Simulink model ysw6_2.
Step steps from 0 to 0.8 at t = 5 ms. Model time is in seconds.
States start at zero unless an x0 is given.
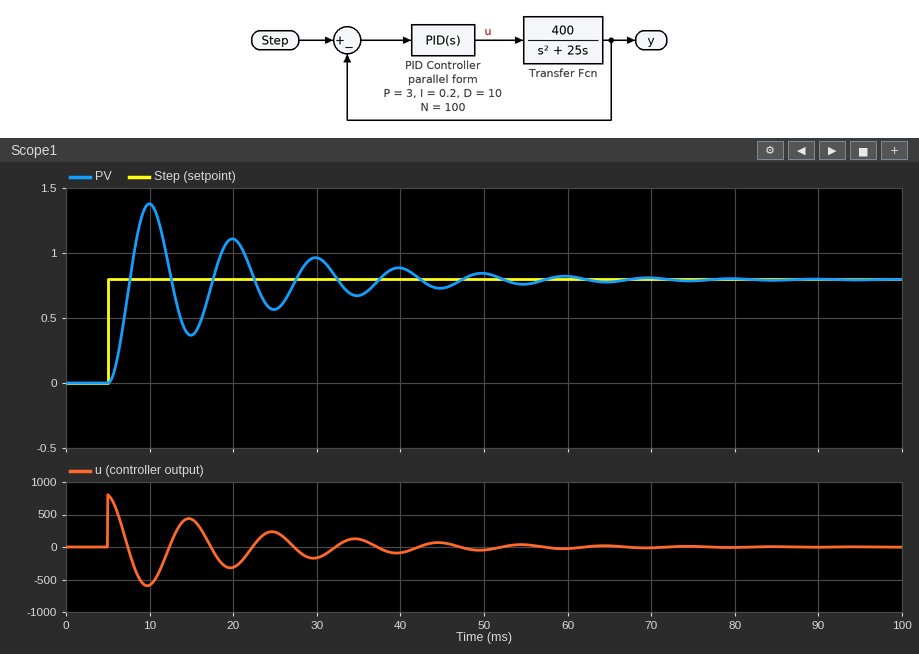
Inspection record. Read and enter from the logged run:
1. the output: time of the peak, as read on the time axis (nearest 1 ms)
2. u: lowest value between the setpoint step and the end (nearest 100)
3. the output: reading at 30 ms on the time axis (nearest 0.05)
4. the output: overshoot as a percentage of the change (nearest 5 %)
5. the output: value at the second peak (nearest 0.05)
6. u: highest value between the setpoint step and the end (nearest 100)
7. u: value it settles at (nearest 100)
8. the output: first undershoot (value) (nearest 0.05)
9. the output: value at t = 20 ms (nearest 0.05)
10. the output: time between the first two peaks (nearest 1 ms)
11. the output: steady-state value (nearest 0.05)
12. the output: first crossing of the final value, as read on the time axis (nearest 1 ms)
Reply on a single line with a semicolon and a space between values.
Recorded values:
10 ms; -600; 0.95; 75 %; 1.10; 800; 0; 0.35; 1.10; 10 ms; 0.80; 8 ms
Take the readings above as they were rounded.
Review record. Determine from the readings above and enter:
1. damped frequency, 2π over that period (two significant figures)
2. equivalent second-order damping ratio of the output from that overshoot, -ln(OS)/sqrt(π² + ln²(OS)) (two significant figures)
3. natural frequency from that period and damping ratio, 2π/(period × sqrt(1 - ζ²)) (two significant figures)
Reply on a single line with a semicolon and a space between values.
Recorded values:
0.63 rad/ms; 0.091; 0.63 rad/ms
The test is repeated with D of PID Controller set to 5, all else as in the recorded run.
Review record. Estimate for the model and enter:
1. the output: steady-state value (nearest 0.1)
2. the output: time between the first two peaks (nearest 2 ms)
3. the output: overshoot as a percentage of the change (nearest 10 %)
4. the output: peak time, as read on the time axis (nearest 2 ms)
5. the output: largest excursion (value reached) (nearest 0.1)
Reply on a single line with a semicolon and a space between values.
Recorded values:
0.8; 14 ms; 60 %; 12 ms; 1.3
